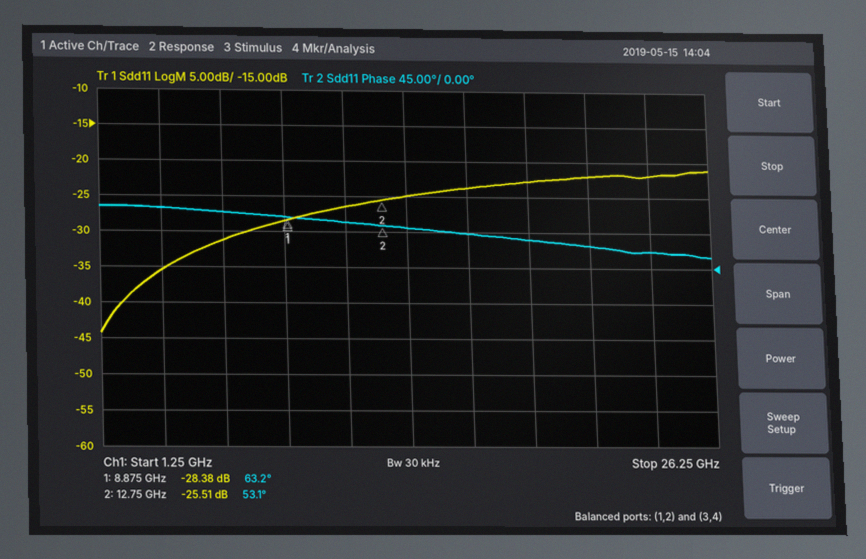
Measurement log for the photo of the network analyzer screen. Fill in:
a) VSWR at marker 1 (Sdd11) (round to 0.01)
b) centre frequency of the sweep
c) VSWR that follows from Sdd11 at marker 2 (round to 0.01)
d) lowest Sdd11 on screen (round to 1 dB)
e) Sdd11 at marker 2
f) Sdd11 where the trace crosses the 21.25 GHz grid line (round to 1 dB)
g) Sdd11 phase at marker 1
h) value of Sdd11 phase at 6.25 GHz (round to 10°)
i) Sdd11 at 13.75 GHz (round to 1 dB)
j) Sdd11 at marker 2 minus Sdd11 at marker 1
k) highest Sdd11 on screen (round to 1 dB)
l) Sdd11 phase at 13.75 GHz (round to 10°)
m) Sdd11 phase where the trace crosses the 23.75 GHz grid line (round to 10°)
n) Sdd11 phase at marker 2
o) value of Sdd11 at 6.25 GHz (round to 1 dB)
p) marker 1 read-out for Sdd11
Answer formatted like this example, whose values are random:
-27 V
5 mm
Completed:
1.08
13.75 GHz
1.11
-44 dB
-25.51 dB
-22 dB
63.2°
70°
-25 dB
2.87 dB
-21 dB
50°
20°
53.1°
-31 dB
-28.38 dB
